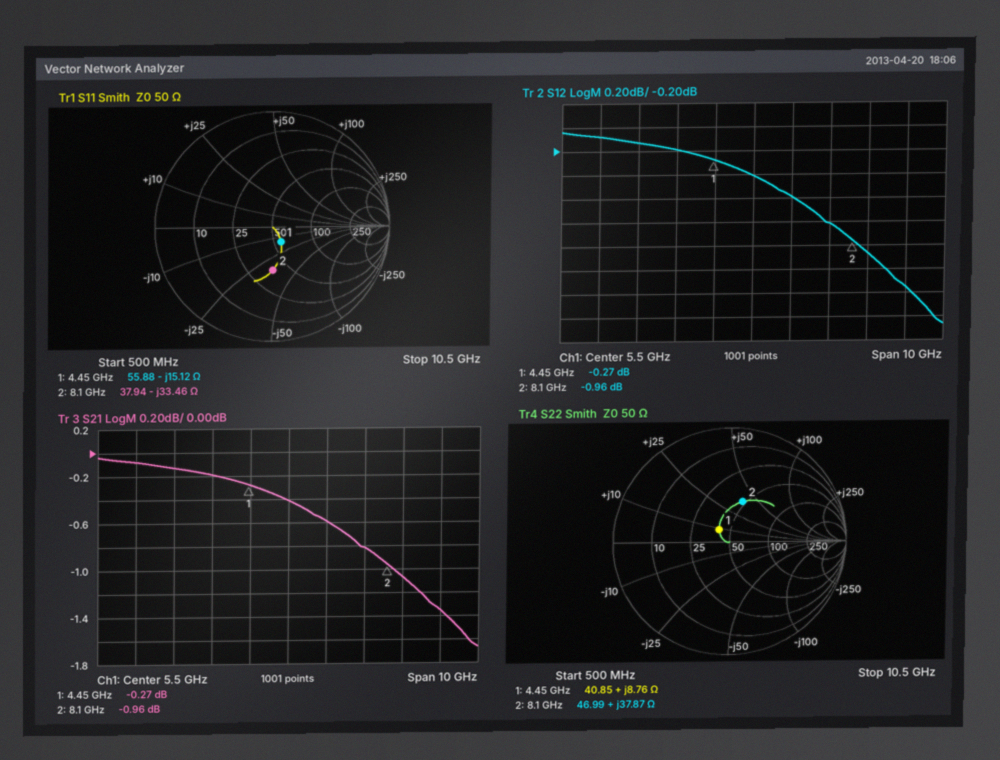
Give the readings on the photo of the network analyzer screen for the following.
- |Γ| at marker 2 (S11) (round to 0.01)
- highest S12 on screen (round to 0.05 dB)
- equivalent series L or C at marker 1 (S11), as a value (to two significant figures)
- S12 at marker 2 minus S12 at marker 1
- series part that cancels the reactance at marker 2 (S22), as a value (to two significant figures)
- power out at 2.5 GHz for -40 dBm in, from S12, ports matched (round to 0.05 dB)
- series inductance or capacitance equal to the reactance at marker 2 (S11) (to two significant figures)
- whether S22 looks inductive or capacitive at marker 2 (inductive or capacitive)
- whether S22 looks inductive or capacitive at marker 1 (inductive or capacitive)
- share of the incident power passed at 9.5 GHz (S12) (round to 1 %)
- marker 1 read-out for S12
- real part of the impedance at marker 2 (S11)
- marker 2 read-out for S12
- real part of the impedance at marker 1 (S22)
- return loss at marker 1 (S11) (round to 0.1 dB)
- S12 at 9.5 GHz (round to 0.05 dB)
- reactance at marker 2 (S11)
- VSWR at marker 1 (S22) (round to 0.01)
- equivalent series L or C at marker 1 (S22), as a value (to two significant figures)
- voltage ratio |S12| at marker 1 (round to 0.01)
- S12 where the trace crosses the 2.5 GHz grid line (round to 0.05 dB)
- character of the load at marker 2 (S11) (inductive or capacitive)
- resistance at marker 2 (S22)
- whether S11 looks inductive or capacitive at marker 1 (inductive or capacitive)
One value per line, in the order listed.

0.38
-0.05 dB
2.4 pF
-0.69 dB
520 fF
-40.15 dBm
590 fF
inductive
inductive
73 %
-0.27 dB
37.94 Ω
-0.96 dB
40.85 Ω
16.4 dB
-1.35 dB
-33.46 Ω
1.32
310 pH
0.97
-0.15 dB
capacitive
46.99 Ω
capacitive
